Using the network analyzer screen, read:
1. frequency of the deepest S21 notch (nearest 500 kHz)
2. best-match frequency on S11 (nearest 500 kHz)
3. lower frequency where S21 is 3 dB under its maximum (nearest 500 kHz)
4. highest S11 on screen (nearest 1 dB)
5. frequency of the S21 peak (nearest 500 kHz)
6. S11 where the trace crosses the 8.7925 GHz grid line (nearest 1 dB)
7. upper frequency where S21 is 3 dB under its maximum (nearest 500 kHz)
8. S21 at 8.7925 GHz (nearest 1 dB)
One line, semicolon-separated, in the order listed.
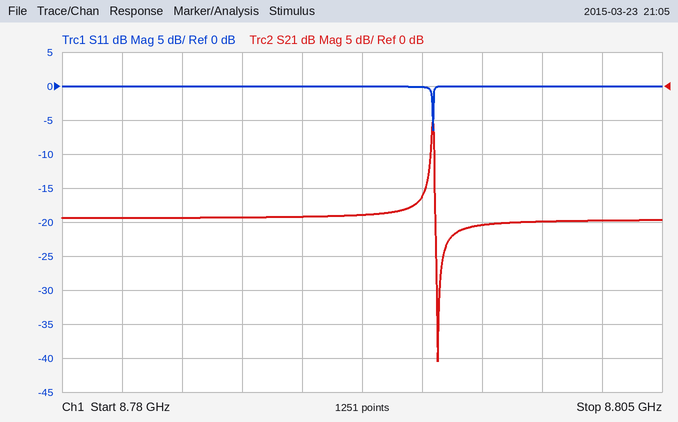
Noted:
8.7955 GHz; 8.7955 GHz; 8.7955 GHz; 0 dB; 8.7955 GHz; 0 dB; 8.7955 GHz; -19 dB
